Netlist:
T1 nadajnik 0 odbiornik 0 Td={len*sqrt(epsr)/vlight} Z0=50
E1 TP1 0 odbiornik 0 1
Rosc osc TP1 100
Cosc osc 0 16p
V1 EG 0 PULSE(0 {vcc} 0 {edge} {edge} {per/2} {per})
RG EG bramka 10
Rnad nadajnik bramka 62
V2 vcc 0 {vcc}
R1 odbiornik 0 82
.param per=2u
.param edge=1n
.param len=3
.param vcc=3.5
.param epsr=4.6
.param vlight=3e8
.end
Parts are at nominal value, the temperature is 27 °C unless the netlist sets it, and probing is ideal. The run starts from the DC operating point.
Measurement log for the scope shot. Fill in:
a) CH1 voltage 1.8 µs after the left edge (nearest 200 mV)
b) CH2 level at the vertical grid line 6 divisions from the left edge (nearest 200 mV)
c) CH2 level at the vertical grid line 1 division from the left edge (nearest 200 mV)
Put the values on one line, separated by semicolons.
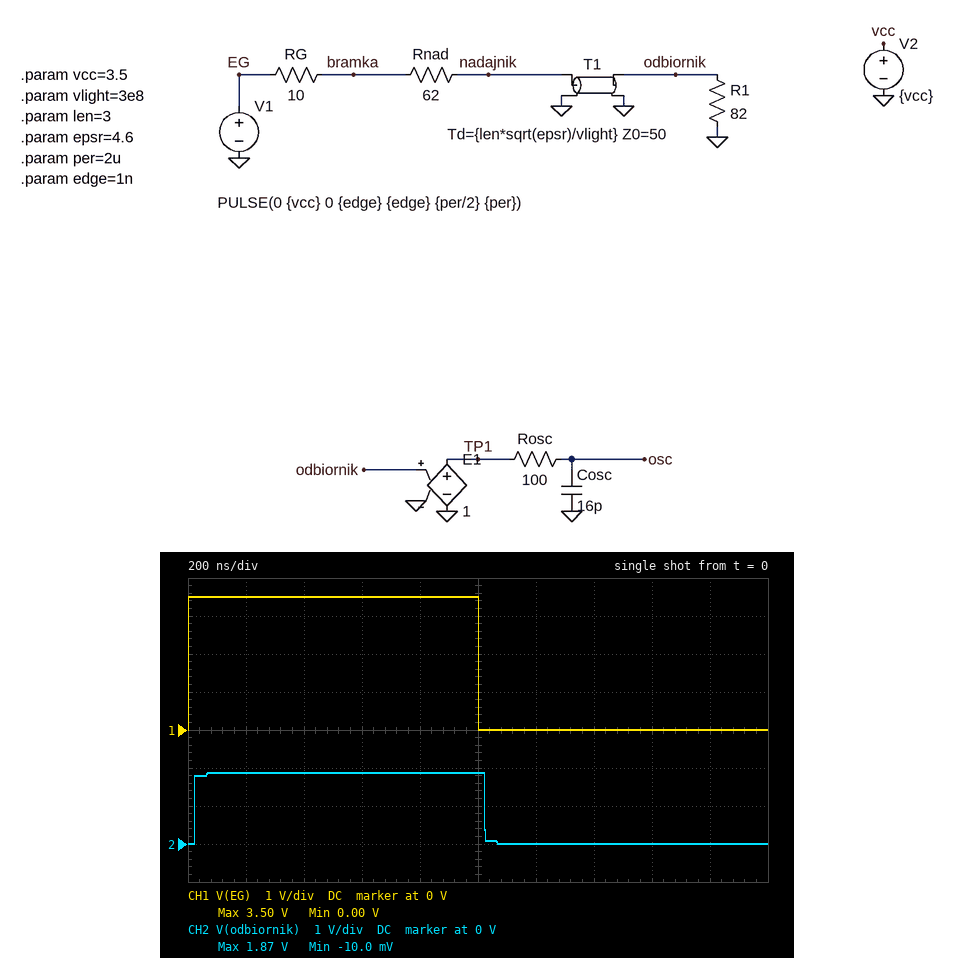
0 V; 0 V; 1.8 V
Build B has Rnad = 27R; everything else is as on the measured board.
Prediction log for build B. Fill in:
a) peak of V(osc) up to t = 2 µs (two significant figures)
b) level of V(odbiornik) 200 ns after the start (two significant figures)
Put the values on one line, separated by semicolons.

2.5 V; 2.4 V
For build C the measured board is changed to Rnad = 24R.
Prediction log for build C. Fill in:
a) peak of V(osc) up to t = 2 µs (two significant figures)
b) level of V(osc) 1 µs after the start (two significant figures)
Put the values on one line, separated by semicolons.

2.6 V; 2.5 V
